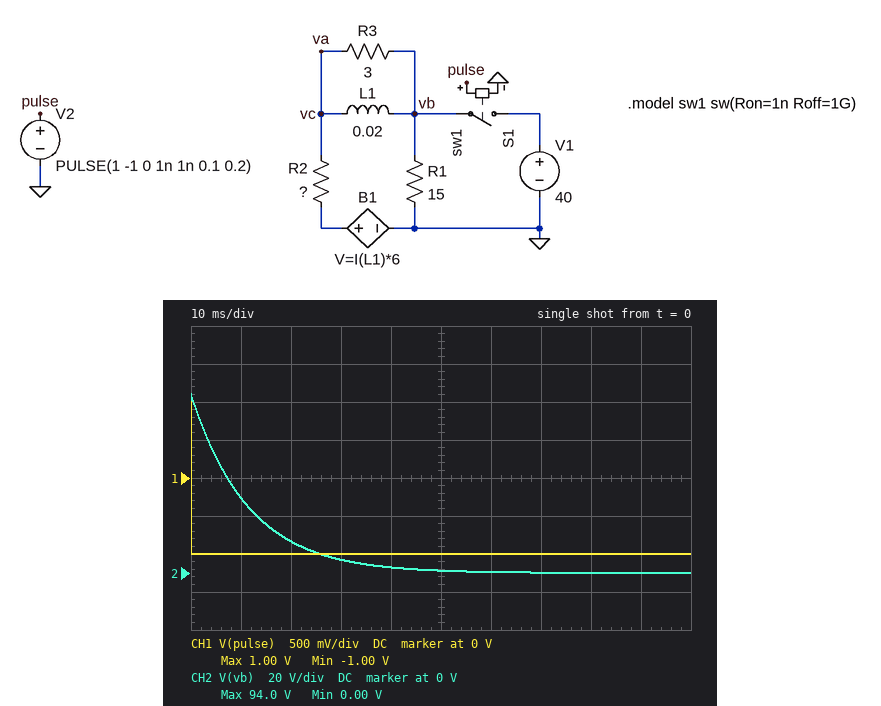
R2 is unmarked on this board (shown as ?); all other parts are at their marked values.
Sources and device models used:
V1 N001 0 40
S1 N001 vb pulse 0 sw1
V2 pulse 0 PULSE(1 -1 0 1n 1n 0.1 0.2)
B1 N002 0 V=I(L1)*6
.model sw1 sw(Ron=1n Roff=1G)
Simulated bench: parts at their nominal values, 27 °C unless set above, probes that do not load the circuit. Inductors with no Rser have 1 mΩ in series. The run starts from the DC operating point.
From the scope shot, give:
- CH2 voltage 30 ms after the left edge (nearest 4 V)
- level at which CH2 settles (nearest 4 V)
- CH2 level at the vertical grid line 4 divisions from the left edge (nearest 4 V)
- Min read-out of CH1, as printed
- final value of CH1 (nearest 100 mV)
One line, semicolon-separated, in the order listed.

8 V; 0 V; 4 V; -1.00 V; -1.0 V
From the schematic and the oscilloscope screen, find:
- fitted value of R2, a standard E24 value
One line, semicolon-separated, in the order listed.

3.3 Ω
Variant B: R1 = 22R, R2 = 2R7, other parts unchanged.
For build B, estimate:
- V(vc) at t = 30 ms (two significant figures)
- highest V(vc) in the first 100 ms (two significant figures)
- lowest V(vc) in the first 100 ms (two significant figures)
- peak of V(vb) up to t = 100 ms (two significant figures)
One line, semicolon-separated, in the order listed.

3.0 V; 62 V; 2.5 mV; 87 V
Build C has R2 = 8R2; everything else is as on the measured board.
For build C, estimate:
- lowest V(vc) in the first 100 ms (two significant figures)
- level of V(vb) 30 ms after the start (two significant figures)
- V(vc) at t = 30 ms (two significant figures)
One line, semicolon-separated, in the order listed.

-58 V; -4.9 V; -3.0 V
